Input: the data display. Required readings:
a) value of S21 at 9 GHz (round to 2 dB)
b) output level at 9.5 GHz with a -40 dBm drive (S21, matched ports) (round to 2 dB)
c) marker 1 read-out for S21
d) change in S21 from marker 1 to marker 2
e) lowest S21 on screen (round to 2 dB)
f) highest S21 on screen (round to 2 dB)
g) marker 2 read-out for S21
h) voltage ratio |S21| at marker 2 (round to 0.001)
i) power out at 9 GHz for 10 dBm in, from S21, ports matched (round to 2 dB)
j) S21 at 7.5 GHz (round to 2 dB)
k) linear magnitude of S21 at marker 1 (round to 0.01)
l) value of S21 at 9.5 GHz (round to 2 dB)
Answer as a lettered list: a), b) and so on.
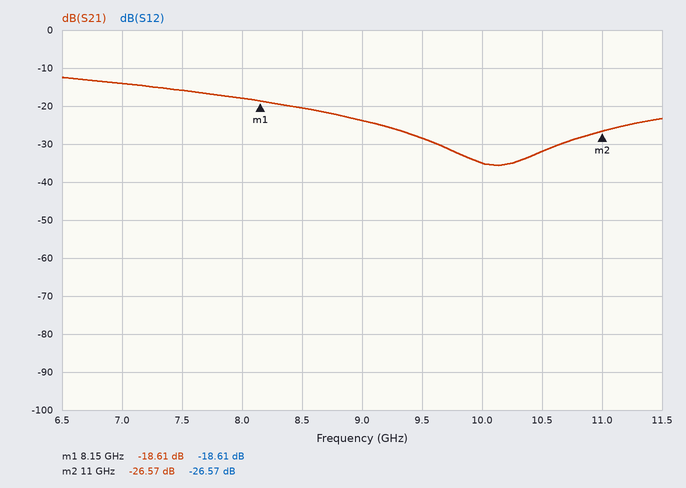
a) -24 dB
b) -68 dBm
c) -18.61 dB
d) -7.96 dB
e) -36 dB
f) -12 dB
g) -26.57 dB
h) 0.047
i) -14 dBm
j) -16 dB
k) 0.12
l) -28 dB
